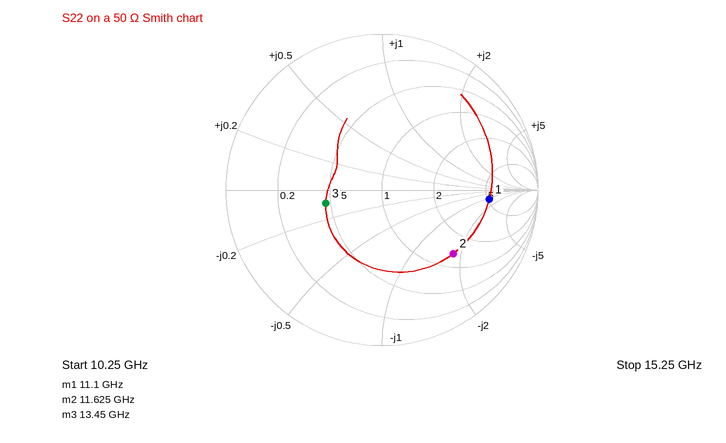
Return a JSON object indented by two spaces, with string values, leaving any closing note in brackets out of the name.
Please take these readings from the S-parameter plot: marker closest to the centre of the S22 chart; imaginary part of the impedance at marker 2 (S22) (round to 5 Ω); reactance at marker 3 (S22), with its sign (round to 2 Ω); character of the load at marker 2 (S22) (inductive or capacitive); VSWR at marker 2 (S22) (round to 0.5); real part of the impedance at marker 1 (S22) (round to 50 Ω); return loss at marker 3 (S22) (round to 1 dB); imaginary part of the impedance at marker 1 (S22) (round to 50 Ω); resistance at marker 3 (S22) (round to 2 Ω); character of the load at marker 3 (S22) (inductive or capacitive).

{
  "marker closest to the centre of the S22 chart": "marker 3",
  "imaginary part of the impedance at marker 2 (S22)": "-90 Ω",
  "reactance at marker 3 (S22), with its sign": "-4 Ω",
  "character of the load at marker 2 (S22)": "capacitive",
  "VSWR at marker 2 (S22)": "4.0",
  "real part of the impedance at marker 1 (S22)": "250 Ω",
  "return loss at marker 3 (S22)": "9 dB",
  "imaginary part of the impedance at marker 1 (S22)": "-50 Ω",
  "resistance at marker 3 (S22)": "24 Ω",
  "character of the load at marker 3 (S22)": "capacitive"
}
